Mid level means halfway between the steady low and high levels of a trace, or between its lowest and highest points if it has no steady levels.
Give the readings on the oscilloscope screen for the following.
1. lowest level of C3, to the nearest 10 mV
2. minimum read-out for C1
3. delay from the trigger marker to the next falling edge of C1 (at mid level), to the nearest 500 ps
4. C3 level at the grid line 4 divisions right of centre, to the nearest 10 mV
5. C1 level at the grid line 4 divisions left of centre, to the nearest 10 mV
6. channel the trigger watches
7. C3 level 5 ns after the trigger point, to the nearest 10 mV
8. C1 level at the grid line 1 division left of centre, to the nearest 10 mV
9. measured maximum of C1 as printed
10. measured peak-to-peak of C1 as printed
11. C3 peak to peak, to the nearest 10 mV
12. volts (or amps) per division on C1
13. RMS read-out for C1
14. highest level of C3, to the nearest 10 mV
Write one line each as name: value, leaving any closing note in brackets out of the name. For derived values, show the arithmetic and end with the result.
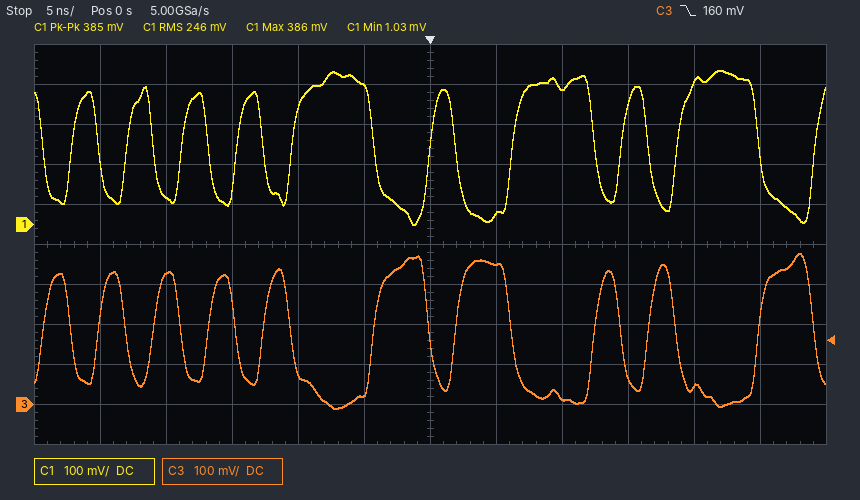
lowest level of C3, to the nearest 10 mV: -10 mV
minimum read-out for C1: 1.03 mV
delay from the trigger marker to the next falling edge of C1 (at mid level), to the nearest 500 ps: 2.0 ns
C3 level at the grid line 4 divisions right of centre, to the nearest 10 mV: 40 mV
C1 level at the grid line 4 divisions left of centre, to the nearest 10 mV: 70 mV
channel the trigger watches: C3
C3 level 5 ns after the trigger point, to the nearest 10 mV: 350 mV
C1 level at the grid line 1 division left of centre, to the nearest 10 mV: 340 mV
measured maximum of C1 as printed: 386 mV
measured peak-to-peak of C1 as printed: 385 mV
C3 peak to peak, to the nearest 10 mV: 380 mV − (-10 mV) = 390 mV
volts (or amps) per division on C1: 100 mV
RMS read-out for C1: 246 mV
highest level of C3, to the nearest 10 mV: 380 mV
